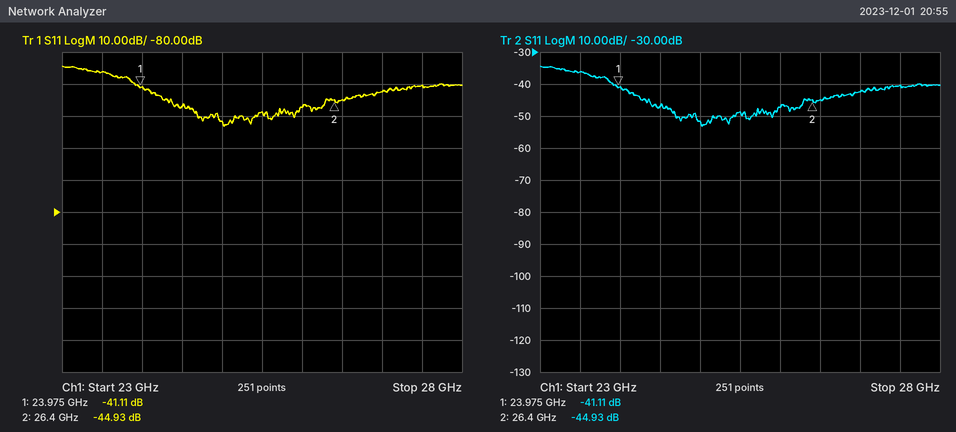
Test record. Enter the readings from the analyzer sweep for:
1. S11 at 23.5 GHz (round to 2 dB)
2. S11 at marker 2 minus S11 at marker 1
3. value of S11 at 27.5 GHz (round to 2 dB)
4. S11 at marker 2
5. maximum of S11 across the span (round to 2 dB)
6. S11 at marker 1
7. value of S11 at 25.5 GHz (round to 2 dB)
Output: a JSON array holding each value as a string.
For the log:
["-36 dB", "-3.82 dB", "-40 dB", "-44.93 dB", "-34 dB", "-41.11 dB", "-48 dB"]
